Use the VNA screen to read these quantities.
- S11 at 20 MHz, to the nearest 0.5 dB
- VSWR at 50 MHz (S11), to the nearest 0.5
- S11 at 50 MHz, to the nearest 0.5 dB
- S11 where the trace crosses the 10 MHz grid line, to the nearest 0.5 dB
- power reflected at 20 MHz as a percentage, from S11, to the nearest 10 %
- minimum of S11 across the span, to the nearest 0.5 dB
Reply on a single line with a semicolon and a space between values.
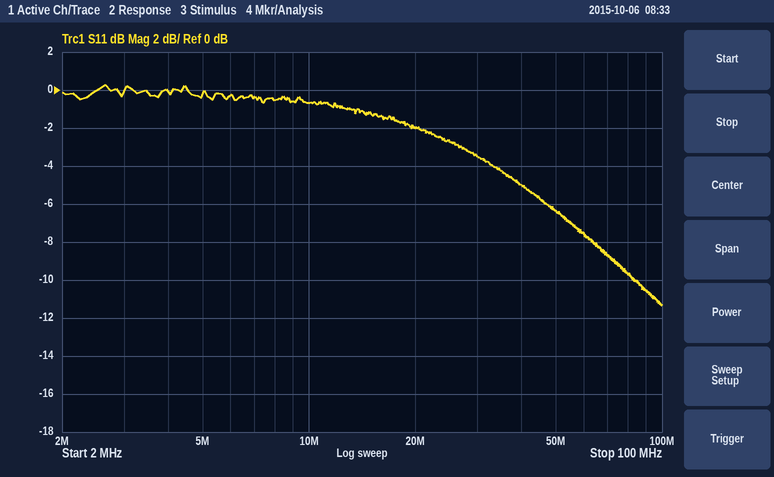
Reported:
-2.0 dB; 3.0; -6.5 dB; -0.5 dB; 60 %; -11.5 dB
